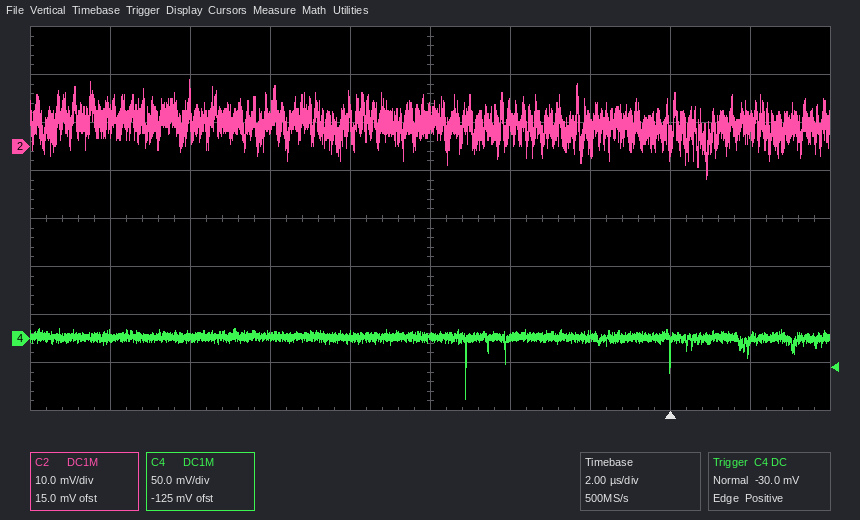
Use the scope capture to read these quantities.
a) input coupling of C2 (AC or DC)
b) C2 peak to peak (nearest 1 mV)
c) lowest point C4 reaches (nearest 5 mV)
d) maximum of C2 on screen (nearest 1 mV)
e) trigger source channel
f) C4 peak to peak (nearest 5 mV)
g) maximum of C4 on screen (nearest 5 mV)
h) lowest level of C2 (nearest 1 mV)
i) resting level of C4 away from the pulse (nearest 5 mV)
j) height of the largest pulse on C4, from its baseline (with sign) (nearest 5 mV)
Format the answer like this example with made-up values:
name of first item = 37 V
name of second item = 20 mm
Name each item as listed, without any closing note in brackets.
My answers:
input coupling of C2 = DC
C2 peak to peak = 21 mV
lowest point C4 reaches = -65 mV
maximum of C2 on screen = 14 mV
trigger source channel = C4
C4 peak to peak = 75 mV
maximum of C4 on screen = 10 mV
lowest level of C2 = -7 mV
resting level of C4 away from the pulse = 0 mV
height of the largest pulse on C4, from its baseline (with sign) = -65 mV
